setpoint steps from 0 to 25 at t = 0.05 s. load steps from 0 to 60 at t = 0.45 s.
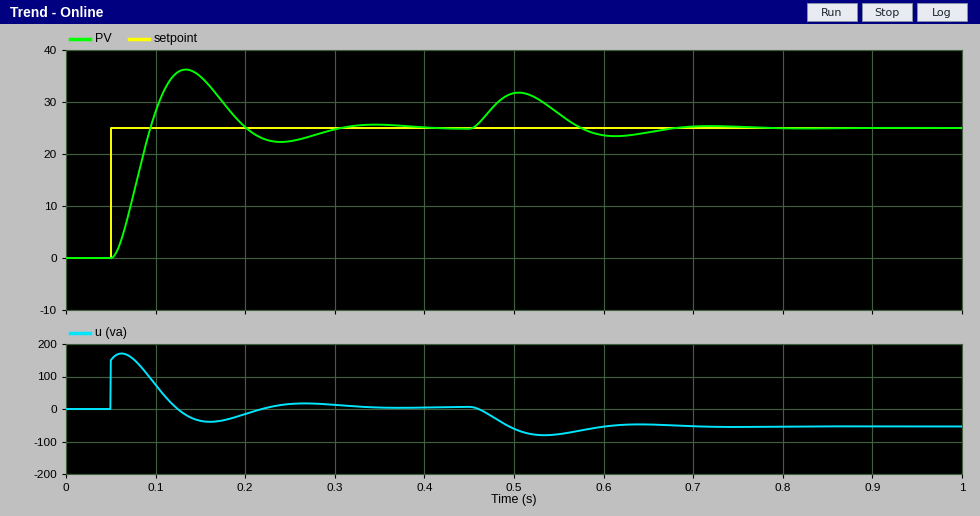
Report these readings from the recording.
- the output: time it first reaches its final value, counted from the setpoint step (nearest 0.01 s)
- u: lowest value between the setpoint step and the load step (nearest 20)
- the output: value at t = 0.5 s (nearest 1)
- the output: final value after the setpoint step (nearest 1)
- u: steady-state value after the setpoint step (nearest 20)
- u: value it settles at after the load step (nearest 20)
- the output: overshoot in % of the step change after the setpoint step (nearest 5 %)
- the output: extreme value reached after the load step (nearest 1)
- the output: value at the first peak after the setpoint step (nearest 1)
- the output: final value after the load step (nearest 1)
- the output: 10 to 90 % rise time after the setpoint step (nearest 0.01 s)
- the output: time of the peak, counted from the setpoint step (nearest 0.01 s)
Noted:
0.04 s
-40
32
25
0
-60
45 %
32
36
25
0.03 s
0.08 s
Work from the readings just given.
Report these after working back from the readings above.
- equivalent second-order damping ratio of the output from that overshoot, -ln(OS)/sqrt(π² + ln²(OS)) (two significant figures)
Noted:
0.25
